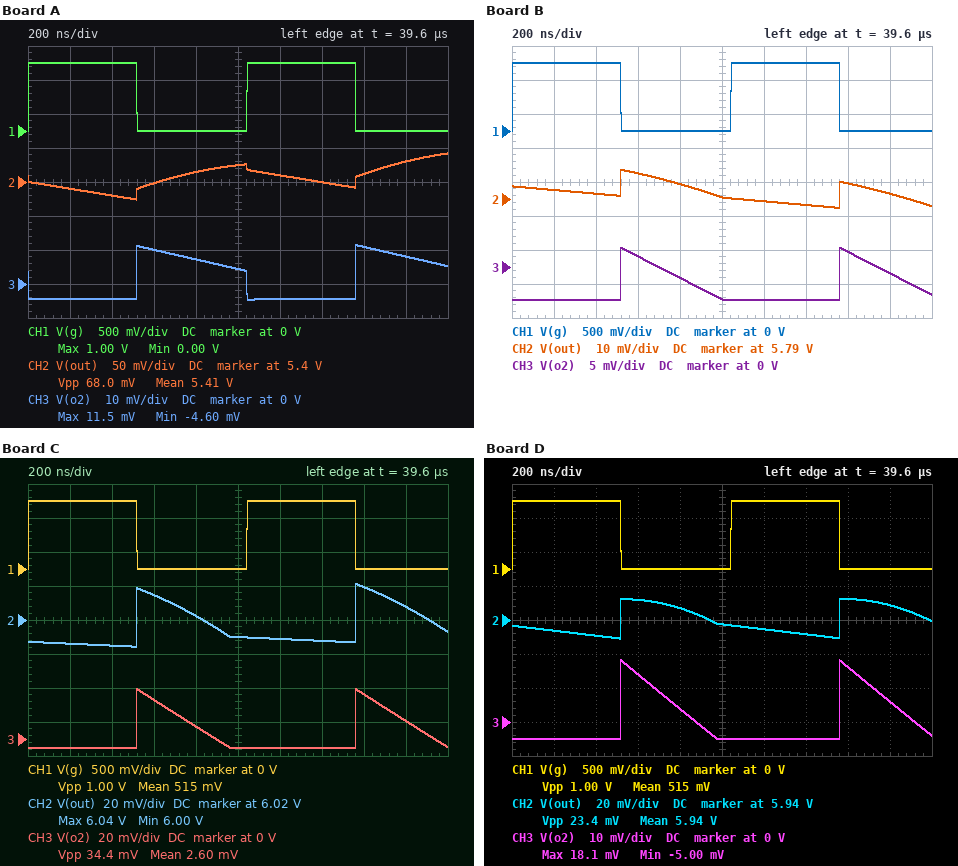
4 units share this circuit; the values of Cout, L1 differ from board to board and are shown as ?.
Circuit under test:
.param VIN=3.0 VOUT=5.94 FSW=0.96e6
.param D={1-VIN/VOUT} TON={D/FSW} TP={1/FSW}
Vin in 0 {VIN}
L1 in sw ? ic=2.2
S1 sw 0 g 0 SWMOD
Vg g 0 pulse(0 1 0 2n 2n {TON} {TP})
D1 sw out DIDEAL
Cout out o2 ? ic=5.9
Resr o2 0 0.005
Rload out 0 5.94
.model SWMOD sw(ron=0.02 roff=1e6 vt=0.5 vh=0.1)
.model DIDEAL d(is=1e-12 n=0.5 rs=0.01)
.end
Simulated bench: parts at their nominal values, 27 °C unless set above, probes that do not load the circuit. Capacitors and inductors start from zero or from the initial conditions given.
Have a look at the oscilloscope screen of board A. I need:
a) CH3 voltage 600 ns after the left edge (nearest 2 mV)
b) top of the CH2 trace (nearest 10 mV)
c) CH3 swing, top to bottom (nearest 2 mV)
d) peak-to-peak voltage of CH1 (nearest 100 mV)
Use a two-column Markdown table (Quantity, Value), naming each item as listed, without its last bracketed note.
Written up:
| Quantity | Value |
|---|---|
| CH3 voltage 600 ns after the left edge | 10 mV |
| top of the CH2 trace | 5.44 V |
| CH3 swing, top to bottom | 16 mV |
| peak-to-peak voltage of CH1 | 1.0 V |
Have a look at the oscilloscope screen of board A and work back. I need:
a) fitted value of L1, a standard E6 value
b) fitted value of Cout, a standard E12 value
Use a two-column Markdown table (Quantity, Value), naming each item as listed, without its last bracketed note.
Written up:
| Quantity | Value |
|---|---|
| fitted value of L1, a standard E6 value | 1 µH |
| fitted value of Cout, a standard E12 value | 18 µF |
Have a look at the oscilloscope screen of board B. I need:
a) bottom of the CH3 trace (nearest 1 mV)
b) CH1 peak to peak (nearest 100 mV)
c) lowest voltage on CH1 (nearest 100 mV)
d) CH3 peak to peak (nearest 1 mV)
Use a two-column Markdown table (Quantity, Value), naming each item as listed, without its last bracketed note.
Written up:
| Quantity | Value |
|---|---|
| bottom of the CH3 trace | -5 mV |
| CH1 peak to peak | 1.0 V |
| lowest voltage on CH1 | 0 V |
| CH3 peak to peak | 8 mV |
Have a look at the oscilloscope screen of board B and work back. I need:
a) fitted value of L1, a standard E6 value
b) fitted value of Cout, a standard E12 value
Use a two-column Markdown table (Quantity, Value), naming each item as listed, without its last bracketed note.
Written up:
| Quantity | Value |
|---|---|
| fitted value of L1, a standard E6 value | 1 µH |
| fitted value of Cout, a standard E12 value | 180 µF |
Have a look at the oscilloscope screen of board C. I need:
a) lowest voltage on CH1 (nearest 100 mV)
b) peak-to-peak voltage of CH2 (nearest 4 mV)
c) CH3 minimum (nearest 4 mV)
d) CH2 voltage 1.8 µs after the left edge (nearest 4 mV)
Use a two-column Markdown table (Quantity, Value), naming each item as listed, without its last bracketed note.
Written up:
| Quantity | Value |
|---|---|
| lowest voltage on CH1 | 0 V |
| peak-to-peak voltage of CH2 | 36 mV |
| CH3 minimum | -4 mV |
| CH2 voltage 1.8 µs after the left edge | 6.028 V |
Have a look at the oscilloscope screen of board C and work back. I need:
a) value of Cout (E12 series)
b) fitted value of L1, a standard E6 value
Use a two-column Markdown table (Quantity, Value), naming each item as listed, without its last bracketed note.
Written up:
| Quantity | Value |
|---|---|
| value of Cout | 180 µF |
| fitted value of L1, a standard E6 value | 220 nH |
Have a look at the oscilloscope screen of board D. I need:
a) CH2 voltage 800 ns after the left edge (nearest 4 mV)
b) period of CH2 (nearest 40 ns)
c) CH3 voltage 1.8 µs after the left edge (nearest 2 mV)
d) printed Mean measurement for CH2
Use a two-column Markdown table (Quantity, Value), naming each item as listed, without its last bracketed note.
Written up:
| Quantity | Value |
|---|---|
| CH2 voltage 800 ns after the left edge | 5.948 V |
| period of CH2 | 1.04 µs |
| CH3 voltage 1.8 µs after the left edge | 6 mV |
| printed Mean measurement for CH2 | 5.94 V |
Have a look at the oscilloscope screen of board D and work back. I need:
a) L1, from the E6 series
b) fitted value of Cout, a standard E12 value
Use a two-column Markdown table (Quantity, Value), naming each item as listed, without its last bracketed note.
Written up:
| Quantity | Value |
|---|---|
| L1, from the E6 series | 330 nH |
| fitted value of Cout, a standard E12 value | 68 µF |
